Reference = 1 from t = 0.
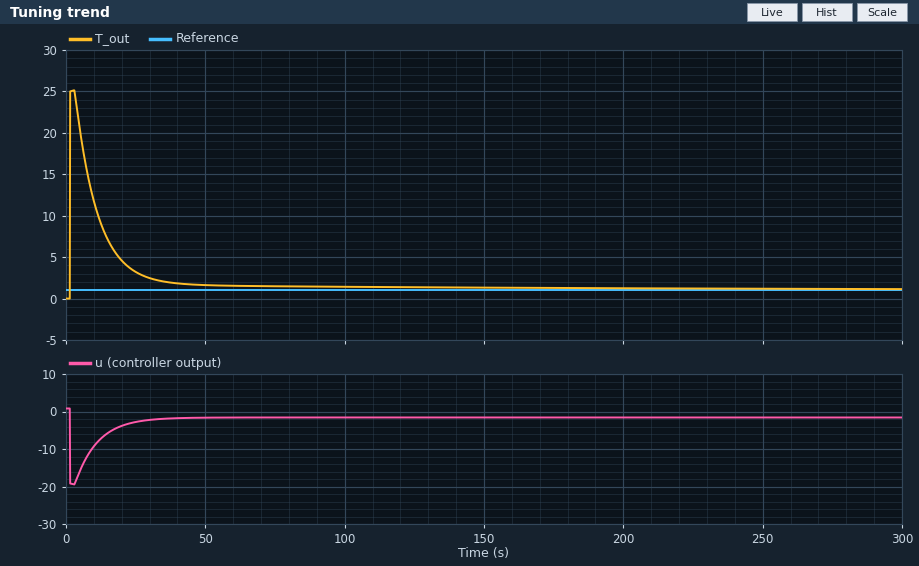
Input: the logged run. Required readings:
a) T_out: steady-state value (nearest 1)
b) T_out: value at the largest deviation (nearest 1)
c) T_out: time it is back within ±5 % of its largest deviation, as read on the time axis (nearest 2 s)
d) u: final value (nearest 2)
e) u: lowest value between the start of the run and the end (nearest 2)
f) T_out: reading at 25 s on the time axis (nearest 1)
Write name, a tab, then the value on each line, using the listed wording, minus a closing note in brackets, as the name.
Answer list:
T_out: steady-state value	1
T_out: value at the largest deviation	25
T_out: time it is back within ±5 % of its largest deviation, as read on the time axis	32 s
u: final value	-2
u: lowest value between the start of the run and the end	-20
T_out: reading at 25 s on the time axis	3
